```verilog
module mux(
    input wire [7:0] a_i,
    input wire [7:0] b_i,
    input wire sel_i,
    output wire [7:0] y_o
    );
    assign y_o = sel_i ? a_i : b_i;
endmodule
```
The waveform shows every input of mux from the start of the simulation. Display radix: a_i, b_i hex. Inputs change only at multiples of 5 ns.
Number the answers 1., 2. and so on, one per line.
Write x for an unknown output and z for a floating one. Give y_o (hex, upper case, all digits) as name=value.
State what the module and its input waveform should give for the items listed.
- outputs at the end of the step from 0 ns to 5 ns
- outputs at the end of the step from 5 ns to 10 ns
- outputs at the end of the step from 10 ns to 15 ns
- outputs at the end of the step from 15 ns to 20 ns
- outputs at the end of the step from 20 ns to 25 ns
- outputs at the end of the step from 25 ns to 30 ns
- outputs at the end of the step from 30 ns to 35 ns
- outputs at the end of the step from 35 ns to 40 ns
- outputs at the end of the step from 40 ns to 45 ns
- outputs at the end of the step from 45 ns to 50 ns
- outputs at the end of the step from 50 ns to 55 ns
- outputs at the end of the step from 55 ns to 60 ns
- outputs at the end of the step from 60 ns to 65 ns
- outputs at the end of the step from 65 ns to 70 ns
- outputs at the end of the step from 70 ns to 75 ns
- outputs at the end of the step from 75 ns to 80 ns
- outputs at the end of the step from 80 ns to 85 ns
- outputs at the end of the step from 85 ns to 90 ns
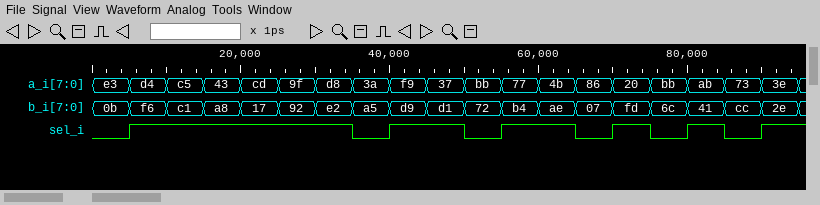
1. y_o=0B
2. y_o=D4
3. y_o=C5
4. y_o=43
5. y_o=CD
6. y_o=9F
7. y_o=D8
8. y_o=A5
9. y_o=F9
10. y_o=37
11. y_o=72
12. y_o=77
13. y_o=4B
14. y_o=07
15. y_o=20
16. y_o=6C
17. y_o=AB
18. y_o=CC
